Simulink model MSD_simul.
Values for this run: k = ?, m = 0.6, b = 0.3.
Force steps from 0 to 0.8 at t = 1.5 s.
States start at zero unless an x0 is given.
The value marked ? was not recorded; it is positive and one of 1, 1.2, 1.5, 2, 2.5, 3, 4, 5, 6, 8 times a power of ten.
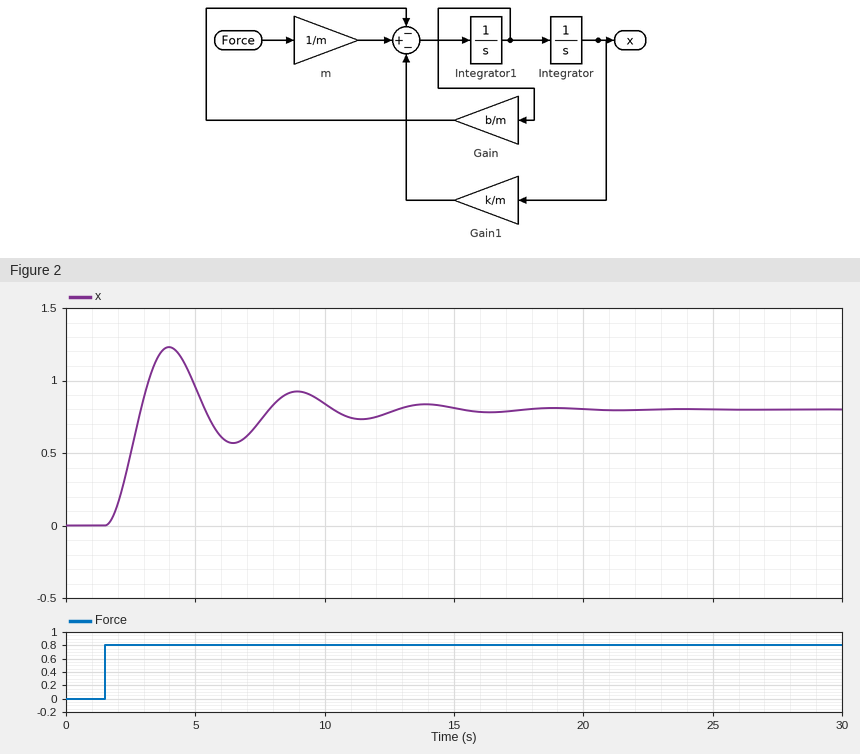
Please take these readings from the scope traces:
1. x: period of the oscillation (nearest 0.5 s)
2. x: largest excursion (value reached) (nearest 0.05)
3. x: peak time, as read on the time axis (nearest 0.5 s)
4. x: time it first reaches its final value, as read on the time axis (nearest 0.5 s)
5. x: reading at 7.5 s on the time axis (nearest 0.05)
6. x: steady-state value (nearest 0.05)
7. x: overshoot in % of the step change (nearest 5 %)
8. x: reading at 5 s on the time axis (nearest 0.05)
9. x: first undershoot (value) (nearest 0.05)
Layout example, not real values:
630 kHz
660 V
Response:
5.0 s
1.25
4.0 s
3.0 s
0.70
0.80
55 %
0.95
0.55
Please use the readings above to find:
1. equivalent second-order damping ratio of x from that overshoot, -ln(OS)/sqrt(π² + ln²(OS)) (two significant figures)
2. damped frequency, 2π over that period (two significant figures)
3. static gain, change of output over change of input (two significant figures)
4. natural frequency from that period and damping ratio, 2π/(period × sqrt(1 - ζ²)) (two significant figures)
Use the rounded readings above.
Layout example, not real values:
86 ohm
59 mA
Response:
0.19
1.3 rad/s
1.0
1.3 rad/s
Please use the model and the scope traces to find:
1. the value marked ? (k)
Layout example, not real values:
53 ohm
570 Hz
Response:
1
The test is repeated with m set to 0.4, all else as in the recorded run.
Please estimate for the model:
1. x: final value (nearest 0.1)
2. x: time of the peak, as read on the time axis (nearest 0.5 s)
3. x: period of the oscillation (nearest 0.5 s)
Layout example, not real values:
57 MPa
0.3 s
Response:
0.8
3.5 s
4.0 s
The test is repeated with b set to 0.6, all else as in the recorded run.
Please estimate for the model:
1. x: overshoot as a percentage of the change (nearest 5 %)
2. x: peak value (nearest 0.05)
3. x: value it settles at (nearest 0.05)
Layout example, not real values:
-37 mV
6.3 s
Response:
25 %
1.00
0.80
